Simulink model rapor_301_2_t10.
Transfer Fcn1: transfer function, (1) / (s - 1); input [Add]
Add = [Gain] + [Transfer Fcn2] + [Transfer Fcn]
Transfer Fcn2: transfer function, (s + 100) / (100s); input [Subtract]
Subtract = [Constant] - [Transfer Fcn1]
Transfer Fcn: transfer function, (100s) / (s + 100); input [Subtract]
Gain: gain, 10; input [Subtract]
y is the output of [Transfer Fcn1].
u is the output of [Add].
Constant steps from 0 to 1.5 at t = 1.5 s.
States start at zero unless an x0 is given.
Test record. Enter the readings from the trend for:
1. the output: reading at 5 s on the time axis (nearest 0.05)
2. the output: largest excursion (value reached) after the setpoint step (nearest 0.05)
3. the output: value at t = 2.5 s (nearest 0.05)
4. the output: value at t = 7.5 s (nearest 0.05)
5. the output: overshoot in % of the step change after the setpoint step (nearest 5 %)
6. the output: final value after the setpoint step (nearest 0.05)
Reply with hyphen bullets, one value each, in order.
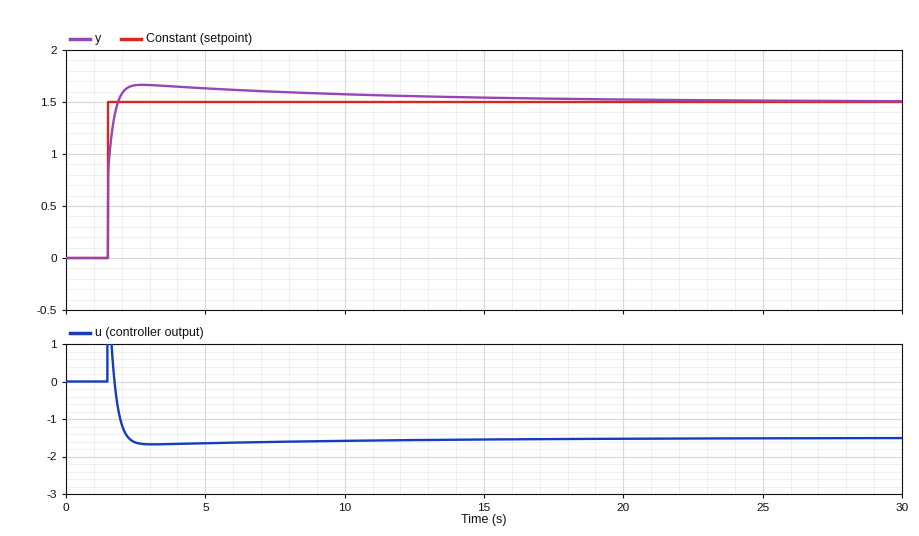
- 1.65
- 1.65
- 1.65
- 1.60
- 10 %
- 1.50
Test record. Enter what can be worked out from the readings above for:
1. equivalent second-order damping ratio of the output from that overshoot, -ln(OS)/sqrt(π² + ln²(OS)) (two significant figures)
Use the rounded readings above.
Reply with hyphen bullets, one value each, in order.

- 0.59
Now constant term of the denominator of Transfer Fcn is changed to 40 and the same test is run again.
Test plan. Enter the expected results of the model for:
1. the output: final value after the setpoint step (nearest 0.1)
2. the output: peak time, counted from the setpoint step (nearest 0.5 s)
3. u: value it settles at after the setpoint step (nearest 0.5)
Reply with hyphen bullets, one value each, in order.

- 1.5
- 2.0 s
- -1.5
